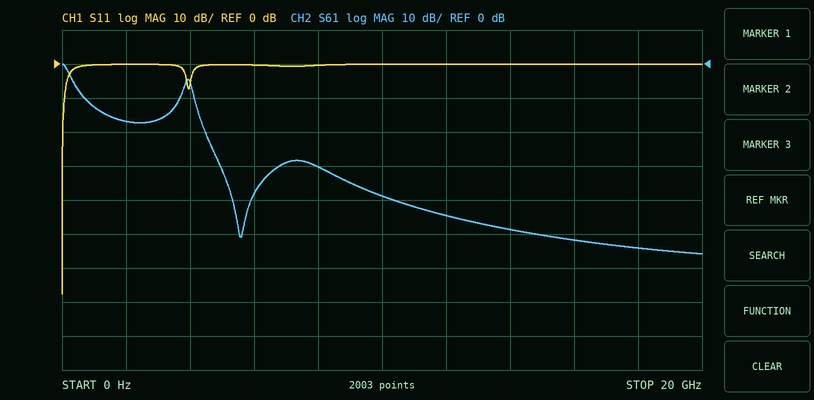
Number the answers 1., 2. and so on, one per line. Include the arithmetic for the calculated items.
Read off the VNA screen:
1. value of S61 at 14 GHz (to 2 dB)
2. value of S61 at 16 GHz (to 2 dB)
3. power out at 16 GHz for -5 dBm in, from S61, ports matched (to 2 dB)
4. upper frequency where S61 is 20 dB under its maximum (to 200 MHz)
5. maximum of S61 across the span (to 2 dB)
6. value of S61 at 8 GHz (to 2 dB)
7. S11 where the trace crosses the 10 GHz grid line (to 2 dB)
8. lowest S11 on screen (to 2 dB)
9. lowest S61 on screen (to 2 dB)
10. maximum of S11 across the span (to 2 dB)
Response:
1. -48 dB
2. -52 dB
3. -5 dBm + (-52 dB) = -56 dBm
4. 4.4 GHz
5. 0 dB
6. -30 dB
7. 0 dB
8. -68 dB
9. -56 dB
10. 0 dB
